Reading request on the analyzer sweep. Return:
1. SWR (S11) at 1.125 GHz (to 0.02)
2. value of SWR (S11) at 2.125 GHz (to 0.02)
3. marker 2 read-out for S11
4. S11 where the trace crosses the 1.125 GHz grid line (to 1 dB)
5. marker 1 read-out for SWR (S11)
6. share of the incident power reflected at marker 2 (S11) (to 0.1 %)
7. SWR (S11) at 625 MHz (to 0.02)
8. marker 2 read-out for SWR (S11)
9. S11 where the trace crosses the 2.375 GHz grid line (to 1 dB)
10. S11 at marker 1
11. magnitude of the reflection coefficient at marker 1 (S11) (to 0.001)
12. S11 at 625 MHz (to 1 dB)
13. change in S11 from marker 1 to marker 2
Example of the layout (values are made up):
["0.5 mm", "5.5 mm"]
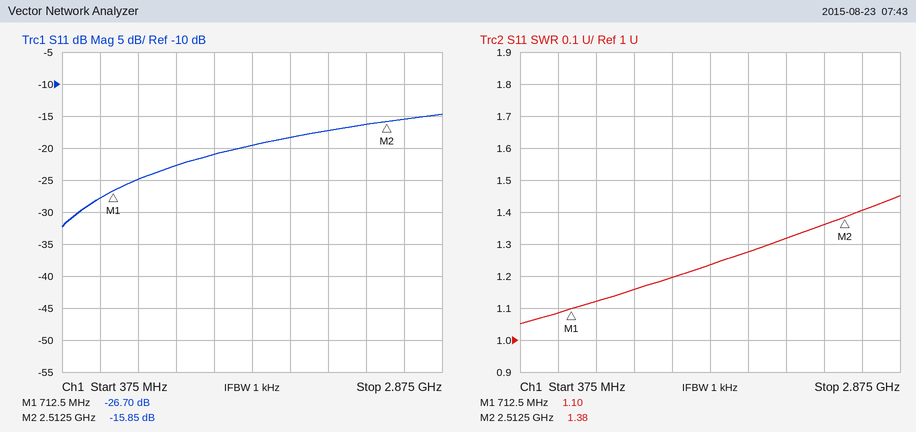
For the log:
["1.16", "1.32", "-15.85 dB", "-23 dB", "1.10", "2.6 %", "1.08", "1.38", "-16 dB", "-26.70 dB", "0.046", "-28 dB", "10.85 dB"]
